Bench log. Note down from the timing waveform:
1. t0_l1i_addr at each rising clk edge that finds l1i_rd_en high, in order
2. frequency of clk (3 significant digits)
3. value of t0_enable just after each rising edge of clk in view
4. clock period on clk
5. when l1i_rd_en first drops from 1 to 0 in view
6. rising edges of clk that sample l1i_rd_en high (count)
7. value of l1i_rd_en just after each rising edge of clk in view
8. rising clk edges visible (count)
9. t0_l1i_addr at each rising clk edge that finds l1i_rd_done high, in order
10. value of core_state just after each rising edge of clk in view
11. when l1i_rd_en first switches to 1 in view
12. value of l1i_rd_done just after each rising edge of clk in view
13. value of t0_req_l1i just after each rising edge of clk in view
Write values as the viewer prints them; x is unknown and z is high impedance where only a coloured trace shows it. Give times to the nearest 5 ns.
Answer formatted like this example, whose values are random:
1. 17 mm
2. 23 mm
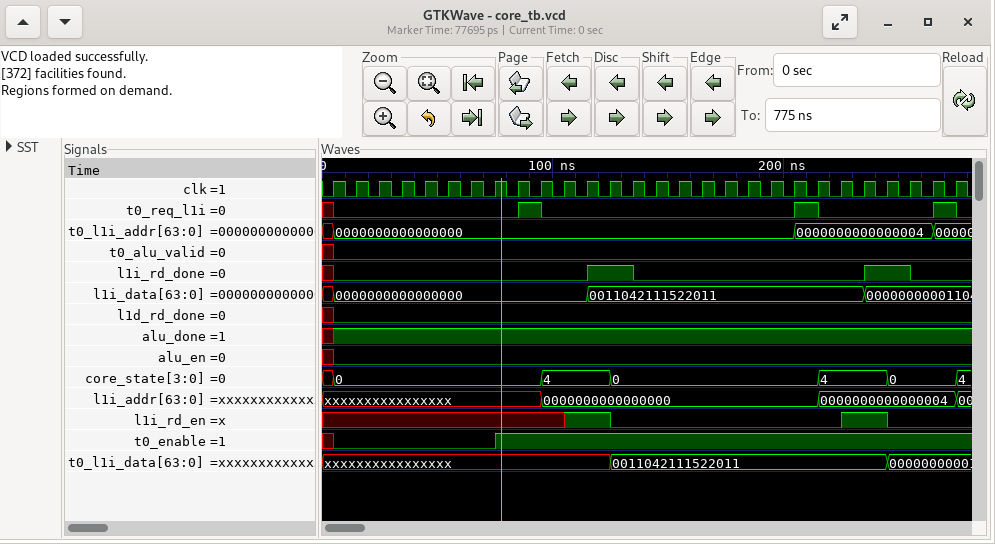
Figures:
1. 0000000000000000, 0000000000000000, 0000000000000004, 0000000000000004
2. 100 MHz
3. 0 0 0 0 0 0 0 1 1 1 1 1 1 1 1 1 1 1 1 1 1 1 1 1 1 1 1 1
4. 10 ns
5. 125 ns
6. 4
7. x x x x x x x x x x 1 1 0 0 0 0 0 0 0 0 0 0 1 1 0 0 0 0
8. 28
9. 0000000000000000, 0000000000000000, 0000000000000004, 0000000000000004
10. 0, 0, 0, 0, 0, 0, 0, 0, 0, 4, 4, 4, 0, 0, 0, 0, 0, 0, 0, 0, 0, 4, 4, 4, 0, 0, 0, 4
11. 105 ns
12. 0 0 0 0 0 0 0 0 0 0 0 1 1 0 0 0 0 0 0 0 0 0 0 1 1 0 0 0
13. 0 0 0 0 0 0 0 0 1 0 0 0 0 0 0 0 0 0 0 0 1 0 0 0 0 0 1 0
